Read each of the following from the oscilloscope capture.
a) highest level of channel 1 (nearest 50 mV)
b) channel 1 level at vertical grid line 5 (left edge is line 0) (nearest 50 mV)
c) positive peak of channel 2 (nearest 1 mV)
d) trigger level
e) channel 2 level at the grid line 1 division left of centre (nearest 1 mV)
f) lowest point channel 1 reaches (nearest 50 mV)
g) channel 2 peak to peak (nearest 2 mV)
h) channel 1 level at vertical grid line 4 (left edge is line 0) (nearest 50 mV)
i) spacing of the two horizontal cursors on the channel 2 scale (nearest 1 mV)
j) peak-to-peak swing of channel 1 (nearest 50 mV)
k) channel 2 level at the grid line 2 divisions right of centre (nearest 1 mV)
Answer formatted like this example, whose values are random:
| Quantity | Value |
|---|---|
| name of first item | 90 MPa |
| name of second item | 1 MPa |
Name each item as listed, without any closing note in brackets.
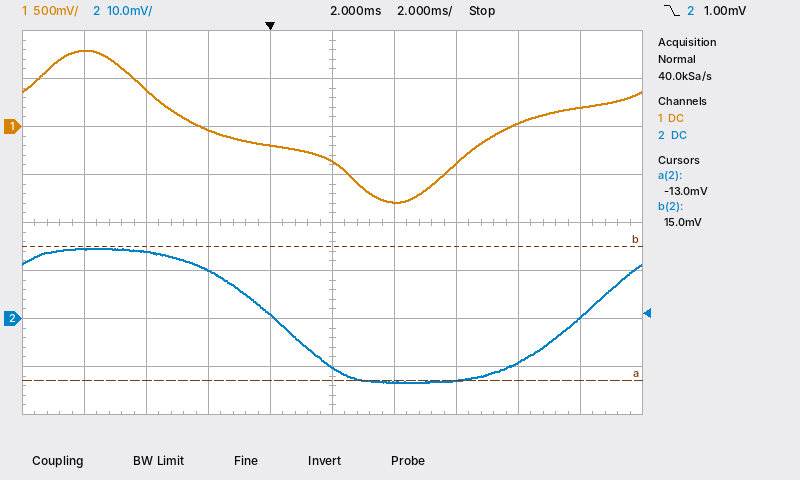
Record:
| Quantity | Value |
|---|---|
| highest level of channel 1 | 800 mV |
| channel 1 level at vertical grid line 5 (left edge is line 0) | -350 mV |
| positive peak of channel 2 | 15 mV |
| trigger level | 1.00 mV |
| channel 2 level at the grid line 1 division left of centre | 1 mV |
| lowest point channel 1 reaches | -800 mV |
| channel 2 peak to peak | 28 mV |
| channel 1 level at vertical grid line 4 (left edge is line 0) | -200 mV |
| spacing of the two horizontal cursors on the channel 2 scale | 28 mV |
| peak-to-peak swing of channel 1 | 1.60 V |
| channel 2 level at the grid line 2 divisions right of centre | -13 mV |
